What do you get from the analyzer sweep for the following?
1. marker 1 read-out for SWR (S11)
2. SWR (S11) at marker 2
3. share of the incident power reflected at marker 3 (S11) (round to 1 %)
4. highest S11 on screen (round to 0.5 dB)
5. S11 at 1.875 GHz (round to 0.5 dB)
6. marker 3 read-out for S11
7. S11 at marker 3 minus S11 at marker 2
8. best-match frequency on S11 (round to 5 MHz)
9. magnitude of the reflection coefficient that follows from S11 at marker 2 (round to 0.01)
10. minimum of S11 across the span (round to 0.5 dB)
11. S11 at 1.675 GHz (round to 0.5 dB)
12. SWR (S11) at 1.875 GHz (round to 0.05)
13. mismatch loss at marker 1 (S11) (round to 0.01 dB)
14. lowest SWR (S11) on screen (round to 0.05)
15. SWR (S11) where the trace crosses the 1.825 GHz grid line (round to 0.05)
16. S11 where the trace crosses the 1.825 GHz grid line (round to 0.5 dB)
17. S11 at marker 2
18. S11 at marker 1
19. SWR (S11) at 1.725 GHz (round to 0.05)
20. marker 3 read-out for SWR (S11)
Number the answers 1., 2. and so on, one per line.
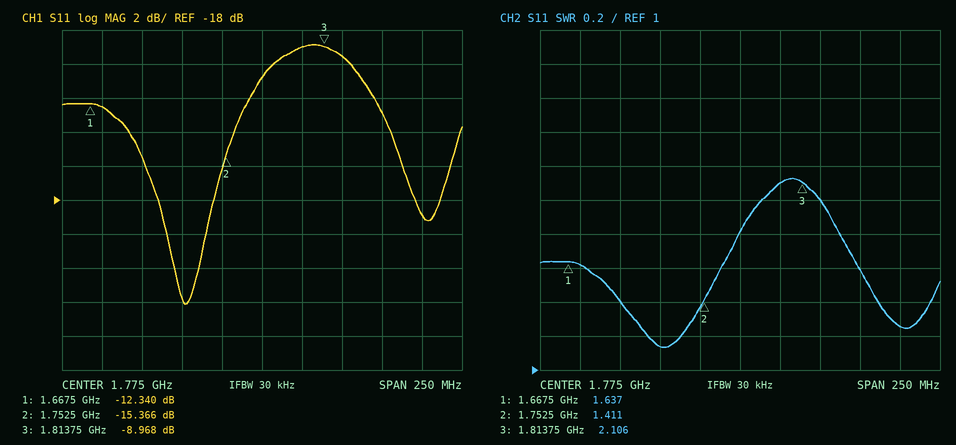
1. 1.637
2. 1.411
3. 13 %
4. -9.0 dB
5. -19.0 dB
6. -8.968 dB
7. 6.398 dB
8. 1.725 GHz
9. 0.17
10. -24.0 dB
11. -12.5 dB
12. 1.25
13. 0.26 dB
14. 1.15
15. 2.00
16. -9.5 dB
17. -15.366 dB
18. -12.340 dB
19. 1.15
20. 2.106
